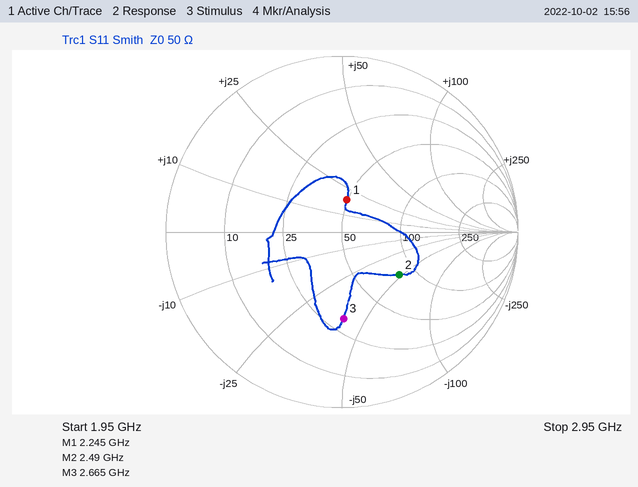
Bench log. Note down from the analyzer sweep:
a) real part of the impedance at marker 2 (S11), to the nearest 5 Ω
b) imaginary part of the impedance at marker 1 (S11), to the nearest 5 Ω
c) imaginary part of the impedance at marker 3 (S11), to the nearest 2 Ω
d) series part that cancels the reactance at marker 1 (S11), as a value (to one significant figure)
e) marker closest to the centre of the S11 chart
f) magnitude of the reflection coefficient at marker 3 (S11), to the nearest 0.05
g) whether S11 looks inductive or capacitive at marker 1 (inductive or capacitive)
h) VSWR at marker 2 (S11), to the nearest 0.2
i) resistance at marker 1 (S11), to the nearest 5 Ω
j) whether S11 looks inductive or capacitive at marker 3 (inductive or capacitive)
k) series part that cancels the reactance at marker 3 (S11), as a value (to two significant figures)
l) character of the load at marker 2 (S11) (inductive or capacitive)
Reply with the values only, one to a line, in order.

80 Ω
+20 Ω
-40 Ω
4 pF
marker 1
0.50
inductive
2.4
50 Ω
capacitive
2.4 nH
capacitive
